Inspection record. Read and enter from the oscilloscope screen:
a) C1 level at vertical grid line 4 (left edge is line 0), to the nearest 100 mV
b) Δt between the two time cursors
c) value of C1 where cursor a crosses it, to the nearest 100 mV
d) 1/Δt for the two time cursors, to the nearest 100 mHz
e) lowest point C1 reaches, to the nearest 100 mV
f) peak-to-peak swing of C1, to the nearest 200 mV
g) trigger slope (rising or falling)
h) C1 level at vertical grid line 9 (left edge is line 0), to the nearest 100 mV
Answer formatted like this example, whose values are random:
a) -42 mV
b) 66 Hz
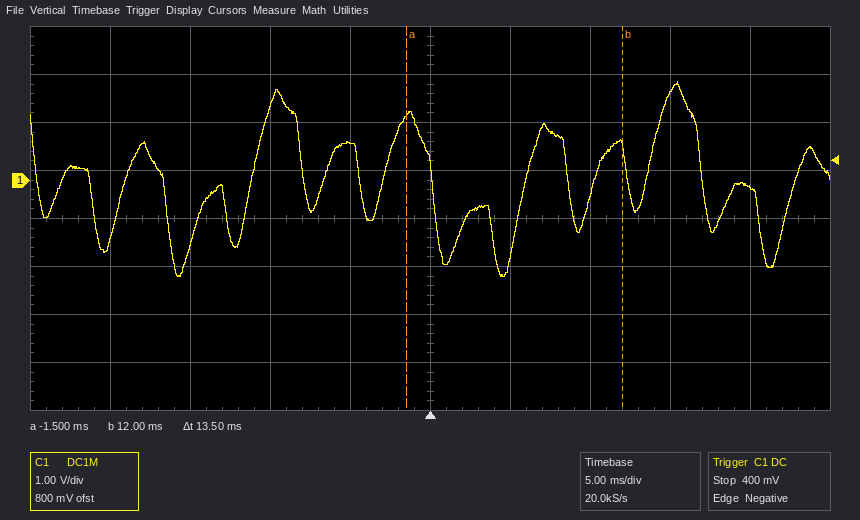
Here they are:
a) 800 mV
b) 13.5 ms
c) 1.3 V
d) 74.1 Hz
e) -2.0 V
f) 4.0 V
g) falling
h) -200 mV
